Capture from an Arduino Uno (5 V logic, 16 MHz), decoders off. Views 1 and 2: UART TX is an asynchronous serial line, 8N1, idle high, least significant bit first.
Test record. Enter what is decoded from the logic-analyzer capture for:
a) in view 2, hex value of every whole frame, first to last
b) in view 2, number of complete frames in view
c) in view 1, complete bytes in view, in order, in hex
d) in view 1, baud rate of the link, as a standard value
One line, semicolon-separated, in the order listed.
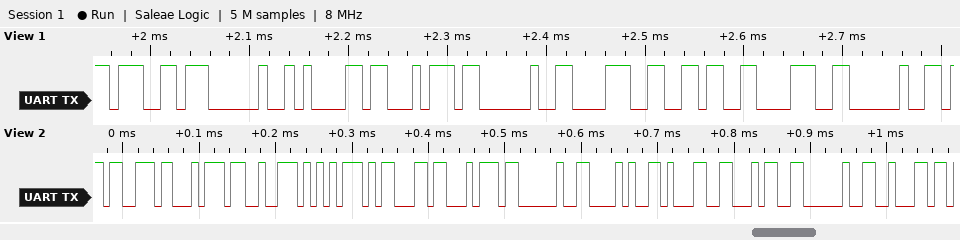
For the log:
73 74 72 75 63 74 20 28 31 34 20 62; 12; 0x67 0x20 0x61 0x74 0x20 0x38 0x36 0x38 0x20; 115200 baud
